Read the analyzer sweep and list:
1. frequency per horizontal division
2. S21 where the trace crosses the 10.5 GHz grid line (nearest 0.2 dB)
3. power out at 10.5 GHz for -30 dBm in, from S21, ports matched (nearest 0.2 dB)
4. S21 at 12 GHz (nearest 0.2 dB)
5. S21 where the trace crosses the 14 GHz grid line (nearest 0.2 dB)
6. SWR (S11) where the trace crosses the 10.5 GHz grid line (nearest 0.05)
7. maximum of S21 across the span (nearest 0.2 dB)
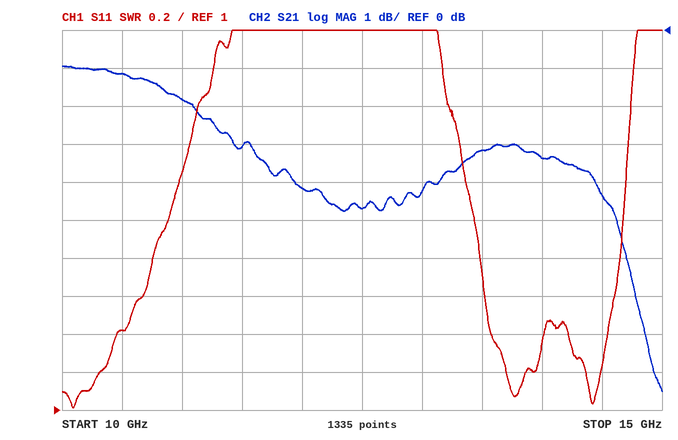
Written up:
500 MHz
-1.2 dB
-31.2 dBm
-4.2 dB
-3.4 dB
1.40
-1.0 dB
